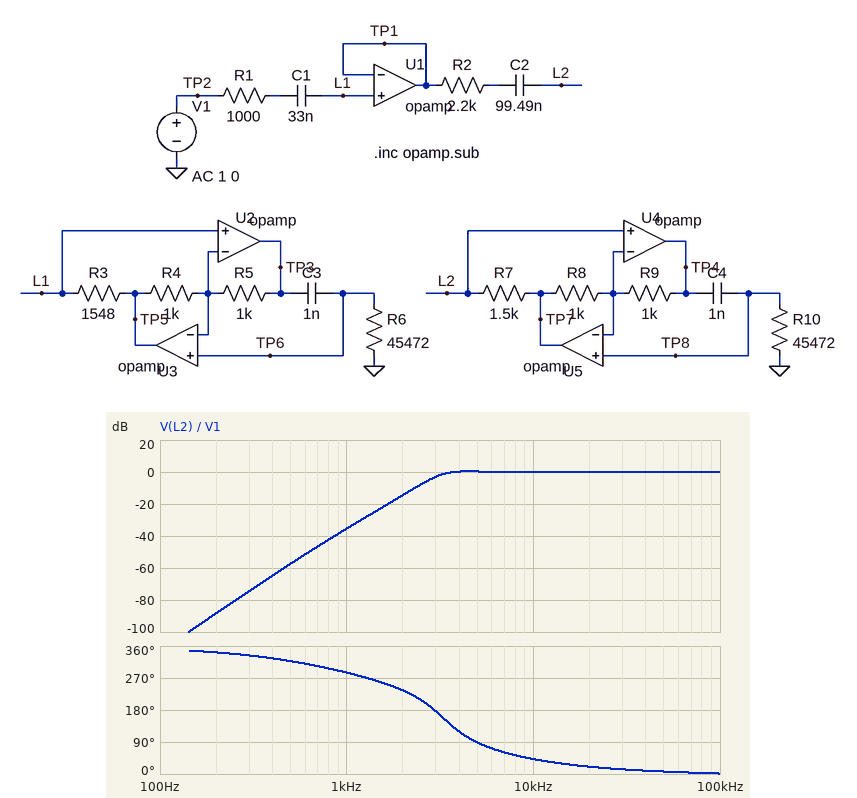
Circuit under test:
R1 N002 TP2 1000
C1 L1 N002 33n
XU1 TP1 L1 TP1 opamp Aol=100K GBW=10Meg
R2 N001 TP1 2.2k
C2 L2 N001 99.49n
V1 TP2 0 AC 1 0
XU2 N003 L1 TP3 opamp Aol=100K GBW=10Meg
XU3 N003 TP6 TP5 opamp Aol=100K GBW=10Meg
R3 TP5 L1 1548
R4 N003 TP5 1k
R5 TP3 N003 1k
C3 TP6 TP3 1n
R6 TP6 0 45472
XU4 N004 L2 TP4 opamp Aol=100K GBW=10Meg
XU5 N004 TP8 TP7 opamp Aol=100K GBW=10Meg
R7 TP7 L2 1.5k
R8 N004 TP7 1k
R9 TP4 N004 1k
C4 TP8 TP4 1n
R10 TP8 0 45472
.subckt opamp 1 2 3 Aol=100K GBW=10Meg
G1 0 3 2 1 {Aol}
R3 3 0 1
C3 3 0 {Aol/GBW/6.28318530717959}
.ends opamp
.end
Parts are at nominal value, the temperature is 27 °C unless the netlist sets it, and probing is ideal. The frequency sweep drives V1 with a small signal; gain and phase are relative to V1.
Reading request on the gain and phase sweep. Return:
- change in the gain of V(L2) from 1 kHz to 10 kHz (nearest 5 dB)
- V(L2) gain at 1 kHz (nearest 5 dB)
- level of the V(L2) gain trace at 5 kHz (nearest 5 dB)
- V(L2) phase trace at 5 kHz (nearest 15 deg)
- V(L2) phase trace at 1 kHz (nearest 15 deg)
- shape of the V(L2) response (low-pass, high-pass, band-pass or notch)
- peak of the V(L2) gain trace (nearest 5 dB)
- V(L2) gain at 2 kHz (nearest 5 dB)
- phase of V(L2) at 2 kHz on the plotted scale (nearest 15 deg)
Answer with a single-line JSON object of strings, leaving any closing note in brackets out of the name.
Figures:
{"change in the gain of V(L2) from 1 kHz to 10 kHz": "35 dB", "V(L2) gain at 1 kHz": "-35 dB", "level of the V(L2) gain trace at 5 kHz": "0 dB", "V(L2) phase trace at 5 kHz": "90 deg", "V(L2) phase trace at 1 kHz": "285 deg", "shape of the V(L2) response": "high-pass", "peak of the V(L2) gain trace": "0 dB", "V(L2) gain at 2 kHz": "-15 dB", "phase of V(L2) at 2 kHz on the plotted scale": "240 deg"}
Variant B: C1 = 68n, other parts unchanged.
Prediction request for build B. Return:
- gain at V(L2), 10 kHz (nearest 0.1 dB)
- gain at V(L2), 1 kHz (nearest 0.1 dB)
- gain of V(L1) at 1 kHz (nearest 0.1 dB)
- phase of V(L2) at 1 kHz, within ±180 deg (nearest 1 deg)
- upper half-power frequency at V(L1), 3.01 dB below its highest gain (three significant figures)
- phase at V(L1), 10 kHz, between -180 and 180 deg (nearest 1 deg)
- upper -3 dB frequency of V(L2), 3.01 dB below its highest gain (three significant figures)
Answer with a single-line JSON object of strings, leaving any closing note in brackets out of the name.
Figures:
{"gain at V(L2), 10 kHz": "-0.5 dB", "gain at V(L2), 1 kHz": "-29.0 dB", "gain of V(L1) at 1 kHz": "-13.7 dB", "phase of V(L2) at 1 kHz, within ±180 deg": "-90 deg", "upper half-power frequency at V(L1), 3.01 dB below its highest gain": "3.13 MHz", "phase at V(L1), 10 kHz, between -180 and 180 deg": "13 deg", "upper -3 dB frequency of V(L2), 3.01 dB below its highest gain": "2.03 MHz"}
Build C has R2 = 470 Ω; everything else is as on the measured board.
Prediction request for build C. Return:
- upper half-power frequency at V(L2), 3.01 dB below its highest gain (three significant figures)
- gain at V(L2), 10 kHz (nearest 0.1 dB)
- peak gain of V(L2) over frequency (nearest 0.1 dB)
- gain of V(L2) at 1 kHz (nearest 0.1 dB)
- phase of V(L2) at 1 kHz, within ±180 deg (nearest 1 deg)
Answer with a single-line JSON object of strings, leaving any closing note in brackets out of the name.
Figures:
{"upper half-power frequency at V(L2), 3.01 dB below its highest gain": "5.76 kHz", "gain at V(L2), 10 kHz": "1.0 dB", "peak gain of V(L2) over frequency": "6.0 dB", "gain of V(L2) at 1 kHz": "-29.5 dB", "phase of V(L2) at 1 kHz, within ±180 deg": "-35 deg"}
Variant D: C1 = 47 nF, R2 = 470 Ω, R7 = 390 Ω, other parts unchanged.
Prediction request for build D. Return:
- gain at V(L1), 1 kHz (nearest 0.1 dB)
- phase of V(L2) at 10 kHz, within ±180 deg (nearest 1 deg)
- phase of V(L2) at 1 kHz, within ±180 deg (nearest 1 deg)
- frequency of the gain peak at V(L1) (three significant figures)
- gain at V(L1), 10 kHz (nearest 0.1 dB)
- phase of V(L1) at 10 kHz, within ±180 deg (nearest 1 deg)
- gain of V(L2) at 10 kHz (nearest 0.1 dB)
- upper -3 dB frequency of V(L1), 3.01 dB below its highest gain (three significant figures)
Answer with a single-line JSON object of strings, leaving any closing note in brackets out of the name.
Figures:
{"gain at V(L1), 1 kHz": "-16.9 dB", "phase of V(L2) at 10 kHz, within ±180 deg": "40 deg", "phase of V(L2) at 1 kHz, within ±180 deg": "-36 deg", "frequency of the gain peak at V(L1)": "3.39 kHz", "gain at V(L1), 10 kHz": "0.4 dB", "phase of V(L1) at 10 kHz, within ±180 deg": "14 deg", "gain of V(L2) at 10 kHz": "0.8 dB", "upper -3 dB frequency of V(L1), 3.01 dB below its highest gain": "1.59 MHz"}
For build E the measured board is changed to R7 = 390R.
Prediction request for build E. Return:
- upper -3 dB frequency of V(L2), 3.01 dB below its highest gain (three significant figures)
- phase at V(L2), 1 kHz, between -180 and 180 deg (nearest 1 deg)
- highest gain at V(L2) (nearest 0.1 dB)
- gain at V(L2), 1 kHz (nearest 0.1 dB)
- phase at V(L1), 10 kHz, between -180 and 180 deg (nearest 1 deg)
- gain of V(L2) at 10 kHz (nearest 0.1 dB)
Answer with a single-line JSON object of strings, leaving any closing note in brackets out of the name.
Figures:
{"upper -3 dB frequency of V(L2), 3.01 dB below its highest gain": "807 kHz", "phase at V(L2), 1 kHz, between -180 and 180 deg": "-69 deg", "highest gain at V(L2)": "0 dB", "gain at V(L2), 1 kHz": "-47.7 dB", "phase at V(L1), 10 kHz, between -180 and 180 deg": "14 deg", "gain of V(L2) at 10 kHz": "-5.9 dB"}
